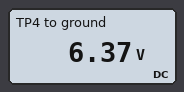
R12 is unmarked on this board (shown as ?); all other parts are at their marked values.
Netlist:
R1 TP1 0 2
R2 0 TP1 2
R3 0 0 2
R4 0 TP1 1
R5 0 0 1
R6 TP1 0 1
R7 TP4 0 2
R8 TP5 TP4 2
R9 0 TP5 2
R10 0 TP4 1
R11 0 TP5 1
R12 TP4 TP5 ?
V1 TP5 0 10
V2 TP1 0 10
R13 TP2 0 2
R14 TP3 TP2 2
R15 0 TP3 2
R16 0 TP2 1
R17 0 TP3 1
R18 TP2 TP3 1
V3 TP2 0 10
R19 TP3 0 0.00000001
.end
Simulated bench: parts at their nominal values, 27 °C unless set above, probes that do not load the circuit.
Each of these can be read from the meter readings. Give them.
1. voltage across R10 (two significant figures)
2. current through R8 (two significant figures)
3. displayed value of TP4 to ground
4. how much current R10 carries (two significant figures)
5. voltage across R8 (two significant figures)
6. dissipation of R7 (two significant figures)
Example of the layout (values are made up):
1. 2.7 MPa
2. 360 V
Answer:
1. 6.4 V
2. 1.8 A
3. 6.37 V
4. 6.4 A
5. 3.6 V
6. 20 W
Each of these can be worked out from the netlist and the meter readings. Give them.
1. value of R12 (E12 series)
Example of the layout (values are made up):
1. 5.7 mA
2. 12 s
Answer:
1. 0.47 Ω
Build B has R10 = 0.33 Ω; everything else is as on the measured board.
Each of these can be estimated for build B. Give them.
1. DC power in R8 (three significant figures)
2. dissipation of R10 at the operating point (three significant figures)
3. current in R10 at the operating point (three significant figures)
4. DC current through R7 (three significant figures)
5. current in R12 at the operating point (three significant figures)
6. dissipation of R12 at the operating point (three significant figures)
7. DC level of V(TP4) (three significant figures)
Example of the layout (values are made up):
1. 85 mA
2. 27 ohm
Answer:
1. 16.4 W
2. 55.2 W
3. 12.9 A
4. 2.13 A
5. 12.2 A
6. 69.9 W
7. 4.27 V
